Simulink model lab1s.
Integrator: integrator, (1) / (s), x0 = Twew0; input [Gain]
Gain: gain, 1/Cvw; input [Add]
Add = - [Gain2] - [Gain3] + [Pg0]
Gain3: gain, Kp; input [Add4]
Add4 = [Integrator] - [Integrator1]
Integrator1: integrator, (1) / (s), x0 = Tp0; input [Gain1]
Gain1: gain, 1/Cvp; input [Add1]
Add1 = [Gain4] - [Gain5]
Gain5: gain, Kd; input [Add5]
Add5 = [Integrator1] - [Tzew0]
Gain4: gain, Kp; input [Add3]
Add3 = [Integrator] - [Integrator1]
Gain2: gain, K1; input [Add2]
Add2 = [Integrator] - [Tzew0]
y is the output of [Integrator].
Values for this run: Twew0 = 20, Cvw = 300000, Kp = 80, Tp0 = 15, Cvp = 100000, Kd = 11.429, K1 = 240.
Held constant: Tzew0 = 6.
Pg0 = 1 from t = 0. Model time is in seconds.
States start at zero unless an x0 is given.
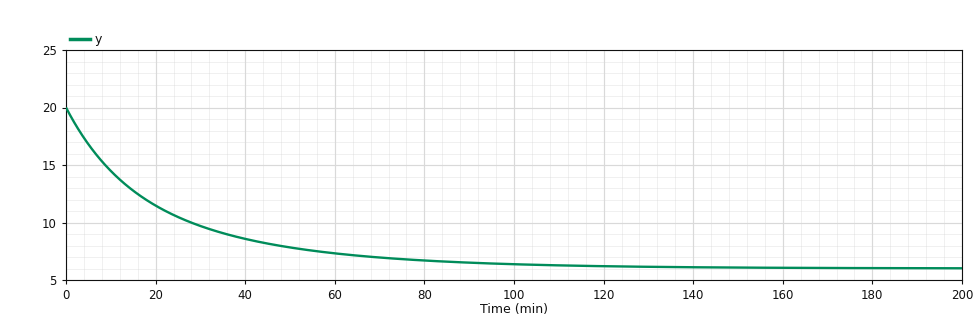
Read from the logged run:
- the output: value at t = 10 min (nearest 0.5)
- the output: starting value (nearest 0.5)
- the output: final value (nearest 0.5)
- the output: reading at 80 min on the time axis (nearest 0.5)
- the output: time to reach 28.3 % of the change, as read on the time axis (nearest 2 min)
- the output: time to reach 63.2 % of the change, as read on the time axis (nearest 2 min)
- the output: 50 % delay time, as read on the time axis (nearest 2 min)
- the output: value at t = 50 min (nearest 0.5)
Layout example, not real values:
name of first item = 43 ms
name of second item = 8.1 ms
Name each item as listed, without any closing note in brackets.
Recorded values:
the output: value at t = 10 min = 14.5
the output: starting value = 20.0
the output: final value = 6.0
the output: reading at 80 min on the time axis = 6.5
the output: time to reach 28.3 % of the change, as read on the time axis = 6 min
the output: time to reach 63.2 % of the change, as read on the time axis = 22 min
the output: 50 % delay time, as read on the time axis = 14 min
the output: value at t = 50 min = 8.0
